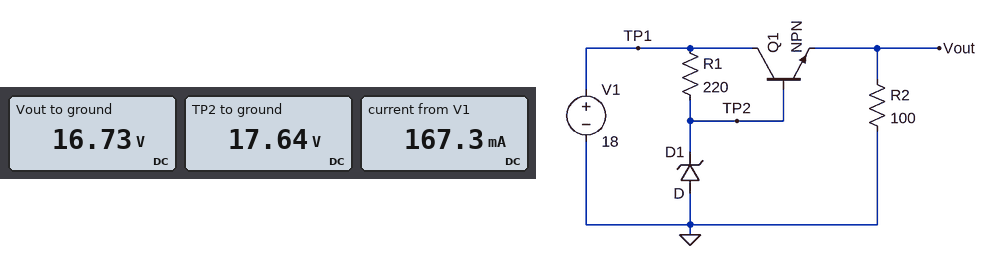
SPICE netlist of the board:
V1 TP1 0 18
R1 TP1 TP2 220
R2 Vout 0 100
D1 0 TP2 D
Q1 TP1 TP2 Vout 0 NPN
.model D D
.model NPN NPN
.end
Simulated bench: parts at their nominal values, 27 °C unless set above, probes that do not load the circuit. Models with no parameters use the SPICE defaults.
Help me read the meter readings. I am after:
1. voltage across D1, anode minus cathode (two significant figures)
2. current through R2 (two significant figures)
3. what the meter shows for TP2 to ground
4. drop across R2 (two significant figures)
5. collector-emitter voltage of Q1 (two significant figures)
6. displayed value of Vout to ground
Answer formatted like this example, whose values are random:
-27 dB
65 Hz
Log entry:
-18 V
170 mA
17.64 V
17 V
1.3 V
16.73 V
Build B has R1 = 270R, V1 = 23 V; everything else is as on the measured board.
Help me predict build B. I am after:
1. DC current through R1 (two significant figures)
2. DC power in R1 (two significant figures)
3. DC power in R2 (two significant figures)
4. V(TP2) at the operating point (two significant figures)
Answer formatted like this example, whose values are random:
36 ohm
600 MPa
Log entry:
2.1 mA
1.2 mW
4.6 W
22 V
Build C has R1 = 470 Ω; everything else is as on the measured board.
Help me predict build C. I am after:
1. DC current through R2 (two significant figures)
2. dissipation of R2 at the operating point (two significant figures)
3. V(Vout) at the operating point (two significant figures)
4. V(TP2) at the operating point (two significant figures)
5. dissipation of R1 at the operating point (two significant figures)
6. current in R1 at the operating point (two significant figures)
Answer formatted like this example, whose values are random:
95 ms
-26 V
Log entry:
160 mA
2.7 W
16 V
17 V
1.2 mW
1.6 mA
